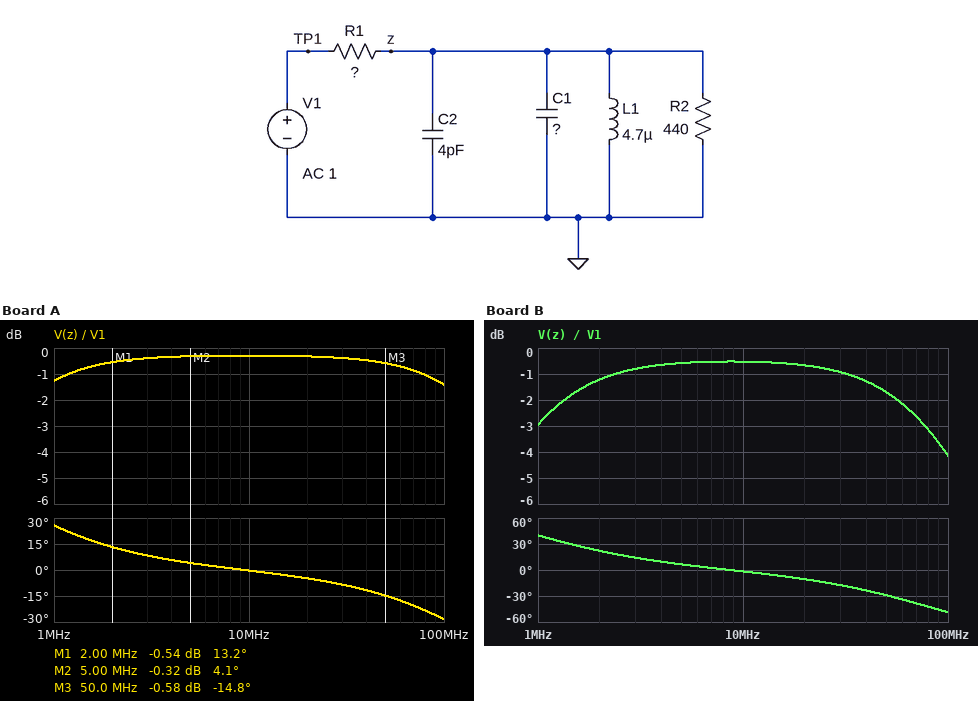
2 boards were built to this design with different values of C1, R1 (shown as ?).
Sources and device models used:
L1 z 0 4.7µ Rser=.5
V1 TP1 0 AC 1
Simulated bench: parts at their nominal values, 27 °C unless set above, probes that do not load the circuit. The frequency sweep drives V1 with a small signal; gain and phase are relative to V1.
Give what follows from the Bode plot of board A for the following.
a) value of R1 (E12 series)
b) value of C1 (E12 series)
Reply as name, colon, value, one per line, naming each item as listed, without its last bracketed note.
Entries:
value of R1: 15 Ω
value of C1: 56 pF
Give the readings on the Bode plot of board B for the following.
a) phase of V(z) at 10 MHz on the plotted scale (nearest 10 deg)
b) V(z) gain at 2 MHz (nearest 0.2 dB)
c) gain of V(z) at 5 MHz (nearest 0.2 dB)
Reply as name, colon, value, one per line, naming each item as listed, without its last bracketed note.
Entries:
phase of V(z) at 10 MHz on the plotted scale: 0 deg
V(z) gain at 2 MHz: -1.2 dB
gain of V(z) at 5 MHz: -0.6 dB
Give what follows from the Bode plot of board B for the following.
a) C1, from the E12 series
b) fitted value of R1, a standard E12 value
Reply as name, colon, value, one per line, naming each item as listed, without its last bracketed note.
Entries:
C1, from the E12 series: 68 pF
fitted value of R1, a standard E12 value: 27 Ω
